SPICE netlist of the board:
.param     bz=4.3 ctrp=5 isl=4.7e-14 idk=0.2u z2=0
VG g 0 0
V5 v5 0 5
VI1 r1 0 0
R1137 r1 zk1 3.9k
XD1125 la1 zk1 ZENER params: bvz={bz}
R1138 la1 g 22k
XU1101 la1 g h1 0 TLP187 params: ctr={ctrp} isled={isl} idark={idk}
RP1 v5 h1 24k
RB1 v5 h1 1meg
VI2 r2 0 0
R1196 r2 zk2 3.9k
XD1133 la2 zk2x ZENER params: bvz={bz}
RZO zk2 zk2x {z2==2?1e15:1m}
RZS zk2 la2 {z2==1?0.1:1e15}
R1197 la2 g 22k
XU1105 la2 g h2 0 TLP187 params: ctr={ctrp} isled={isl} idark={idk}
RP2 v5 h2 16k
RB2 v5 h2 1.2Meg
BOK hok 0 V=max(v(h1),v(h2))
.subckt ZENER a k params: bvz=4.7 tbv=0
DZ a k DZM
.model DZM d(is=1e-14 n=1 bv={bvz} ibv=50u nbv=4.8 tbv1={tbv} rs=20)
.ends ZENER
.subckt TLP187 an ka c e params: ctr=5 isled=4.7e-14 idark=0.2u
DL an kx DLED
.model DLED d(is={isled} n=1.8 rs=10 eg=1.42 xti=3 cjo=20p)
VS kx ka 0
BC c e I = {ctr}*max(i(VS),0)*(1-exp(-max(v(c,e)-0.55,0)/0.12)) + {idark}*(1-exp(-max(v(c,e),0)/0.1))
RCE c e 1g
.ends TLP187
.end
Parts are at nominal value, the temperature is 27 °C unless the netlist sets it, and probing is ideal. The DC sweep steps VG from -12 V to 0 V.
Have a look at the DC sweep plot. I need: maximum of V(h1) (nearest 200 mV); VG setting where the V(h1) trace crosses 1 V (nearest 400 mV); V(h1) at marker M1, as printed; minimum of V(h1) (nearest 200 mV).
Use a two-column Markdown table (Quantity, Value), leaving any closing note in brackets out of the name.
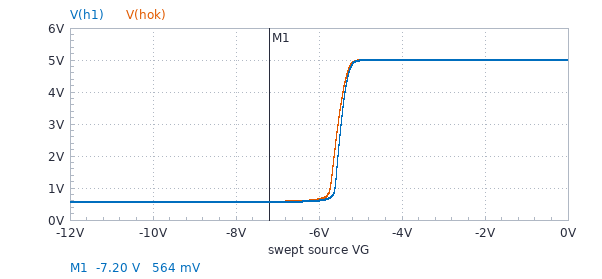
| Quantity | Value |
|---|---|
| maximum of V(h1) | 5.0 V |
| VG setting where the V(h1) trace crosses 1 V | -5.6 V |
| V(h1) at marker M1, as printed | 564 mV |
| minimum of V(h1) | 600 mV |
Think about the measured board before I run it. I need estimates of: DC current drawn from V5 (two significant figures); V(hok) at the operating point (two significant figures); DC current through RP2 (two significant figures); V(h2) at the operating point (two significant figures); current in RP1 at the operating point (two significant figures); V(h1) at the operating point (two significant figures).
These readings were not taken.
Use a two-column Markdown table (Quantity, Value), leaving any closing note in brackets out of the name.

| Quantity | Value |
|---|---|
| DC current drawn from V5 | 410 nA |
| V(hok) at the operating point | 5.0 V |
| DC current through RP2 | 200 nA |
| V(h2) at the operating point | 5.0 V |
| current in RP1 at the operating point | 200 nA |
| V(h1) at the operating point | 5.0 V |
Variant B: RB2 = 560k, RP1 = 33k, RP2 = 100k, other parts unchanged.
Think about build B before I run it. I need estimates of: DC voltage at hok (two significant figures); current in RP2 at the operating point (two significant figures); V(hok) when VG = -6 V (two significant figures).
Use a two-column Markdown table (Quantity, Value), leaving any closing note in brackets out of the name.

| Quantity | Value |
|---|---|
| DC voltage at hok | 5.0 V |
| current in RP2 at the operating point | 170 nA |
| V(hok) when VG = -6 V | 590 mV |
